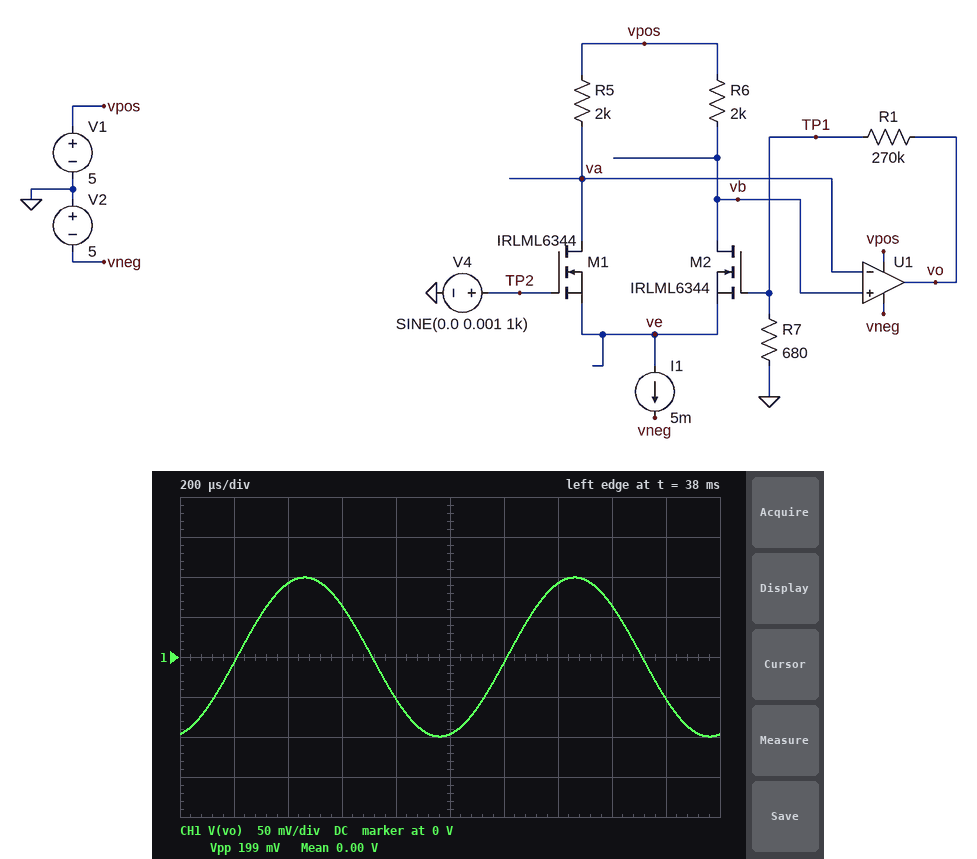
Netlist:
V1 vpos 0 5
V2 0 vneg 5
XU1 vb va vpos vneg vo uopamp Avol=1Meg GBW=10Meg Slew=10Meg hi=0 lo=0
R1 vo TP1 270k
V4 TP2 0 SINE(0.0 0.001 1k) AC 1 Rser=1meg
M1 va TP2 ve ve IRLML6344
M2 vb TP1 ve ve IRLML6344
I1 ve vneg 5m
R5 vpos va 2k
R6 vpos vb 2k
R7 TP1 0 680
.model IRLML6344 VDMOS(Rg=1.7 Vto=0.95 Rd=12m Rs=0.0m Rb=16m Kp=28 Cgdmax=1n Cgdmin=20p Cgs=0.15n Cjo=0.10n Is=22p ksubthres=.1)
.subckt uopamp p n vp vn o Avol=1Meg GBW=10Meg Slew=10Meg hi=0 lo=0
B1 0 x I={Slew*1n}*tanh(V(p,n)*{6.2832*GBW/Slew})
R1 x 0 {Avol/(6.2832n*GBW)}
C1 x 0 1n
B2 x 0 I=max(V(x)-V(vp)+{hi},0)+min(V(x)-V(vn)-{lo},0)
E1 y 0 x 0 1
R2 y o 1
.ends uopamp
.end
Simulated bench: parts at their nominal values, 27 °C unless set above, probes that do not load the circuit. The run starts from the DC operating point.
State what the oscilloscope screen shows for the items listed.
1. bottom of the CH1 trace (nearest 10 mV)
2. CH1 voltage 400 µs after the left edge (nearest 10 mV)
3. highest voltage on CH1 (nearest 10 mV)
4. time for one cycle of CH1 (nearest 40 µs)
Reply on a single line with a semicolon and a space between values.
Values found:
-100 mV; 90 mV; 100 mV; 1.00 ms
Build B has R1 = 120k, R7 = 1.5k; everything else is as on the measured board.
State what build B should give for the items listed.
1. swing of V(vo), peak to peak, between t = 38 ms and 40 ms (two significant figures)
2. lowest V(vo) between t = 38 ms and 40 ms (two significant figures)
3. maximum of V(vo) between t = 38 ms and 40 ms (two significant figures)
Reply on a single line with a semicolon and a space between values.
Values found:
40 mV; -20 mV; 20 mV
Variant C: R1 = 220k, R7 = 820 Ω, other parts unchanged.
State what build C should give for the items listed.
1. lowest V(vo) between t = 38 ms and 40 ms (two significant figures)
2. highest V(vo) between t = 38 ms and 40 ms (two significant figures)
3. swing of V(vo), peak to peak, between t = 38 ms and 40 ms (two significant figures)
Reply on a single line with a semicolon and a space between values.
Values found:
-67 mV; 67 mV; 130 mV
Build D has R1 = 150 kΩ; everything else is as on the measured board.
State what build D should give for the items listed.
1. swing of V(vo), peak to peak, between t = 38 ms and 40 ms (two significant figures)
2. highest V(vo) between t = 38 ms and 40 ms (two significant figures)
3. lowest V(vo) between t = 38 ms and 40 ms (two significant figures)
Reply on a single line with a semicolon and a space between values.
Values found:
110 mV; 55 mV; -55 mV
